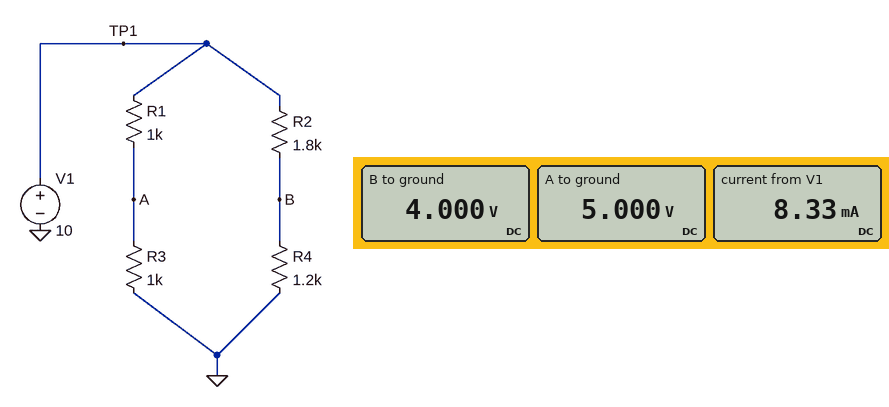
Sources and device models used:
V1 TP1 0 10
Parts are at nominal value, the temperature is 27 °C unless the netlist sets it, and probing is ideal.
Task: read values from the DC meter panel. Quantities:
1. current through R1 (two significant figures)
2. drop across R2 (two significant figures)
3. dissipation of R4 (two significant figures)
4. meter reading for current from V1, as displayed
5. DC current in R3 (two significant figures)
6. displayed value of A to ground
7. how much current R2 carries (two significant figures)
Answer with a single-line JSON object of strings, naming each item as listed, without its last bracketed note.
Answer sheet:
{"current through R1": "5.0 mA", "drop across R2": "6.0 V", "dissipation of R4": "13 mW", "meter reading for current from V1, as displayed": "8.33 mA", "DC current in R3": "5.0 mA", "displayed value of A to ground": "5.000 V", "how much current R2 carries": "3.3 mA"}
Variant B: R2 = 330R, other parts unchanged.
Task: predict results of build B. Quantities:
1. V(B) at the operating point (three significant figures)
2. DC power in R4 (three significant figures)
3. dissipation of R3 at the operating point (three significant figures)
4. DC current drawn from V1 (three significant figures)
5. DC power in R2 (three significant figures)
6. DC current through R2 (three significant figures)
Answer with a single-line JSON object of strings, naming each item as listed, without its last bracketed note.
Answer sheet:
{"V(B) at the operating point": "7.84 V", "DC power in R4": "51.3 mW", "dissipation of R3 at the operating point": "25.0 mW", "DC current drawn from V1": "11.5 mA", "DC power in R2": "14.1 mW", "DC current through R2": "6.54 mA"}
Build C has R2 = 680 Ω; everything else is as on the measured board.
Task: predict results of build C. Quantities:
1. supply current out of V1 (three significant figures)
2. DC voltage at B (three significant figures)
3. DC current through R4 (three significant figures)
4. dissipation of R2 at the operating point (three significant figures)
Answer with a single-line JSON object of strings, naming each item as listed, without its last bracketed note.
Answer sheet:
{"supply current out of V1": "10.3 mA", "DC voltage at B": "6.38 V", "DC current through R4": "5.32 mA", "dissipation of R2 at the operating point": "19.2 mW"}
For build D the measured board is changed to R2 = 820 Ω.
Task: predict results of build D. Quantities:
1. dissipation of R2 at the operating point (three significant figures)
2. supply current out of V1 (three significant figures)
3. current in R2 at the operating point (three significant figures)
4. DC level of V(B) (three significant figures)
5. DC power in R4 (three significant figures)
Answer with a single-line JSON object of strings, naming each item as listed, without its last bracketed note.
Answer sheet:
{"dissipation of R2 at the operating point": "20.1 mW", "supply current out of V1": "9.95 mA", "current in R2 at the operating point": "4.95 mA", "DC level of V(B)": "5.94 V", "DC power in R4": "29.4 mW"}
